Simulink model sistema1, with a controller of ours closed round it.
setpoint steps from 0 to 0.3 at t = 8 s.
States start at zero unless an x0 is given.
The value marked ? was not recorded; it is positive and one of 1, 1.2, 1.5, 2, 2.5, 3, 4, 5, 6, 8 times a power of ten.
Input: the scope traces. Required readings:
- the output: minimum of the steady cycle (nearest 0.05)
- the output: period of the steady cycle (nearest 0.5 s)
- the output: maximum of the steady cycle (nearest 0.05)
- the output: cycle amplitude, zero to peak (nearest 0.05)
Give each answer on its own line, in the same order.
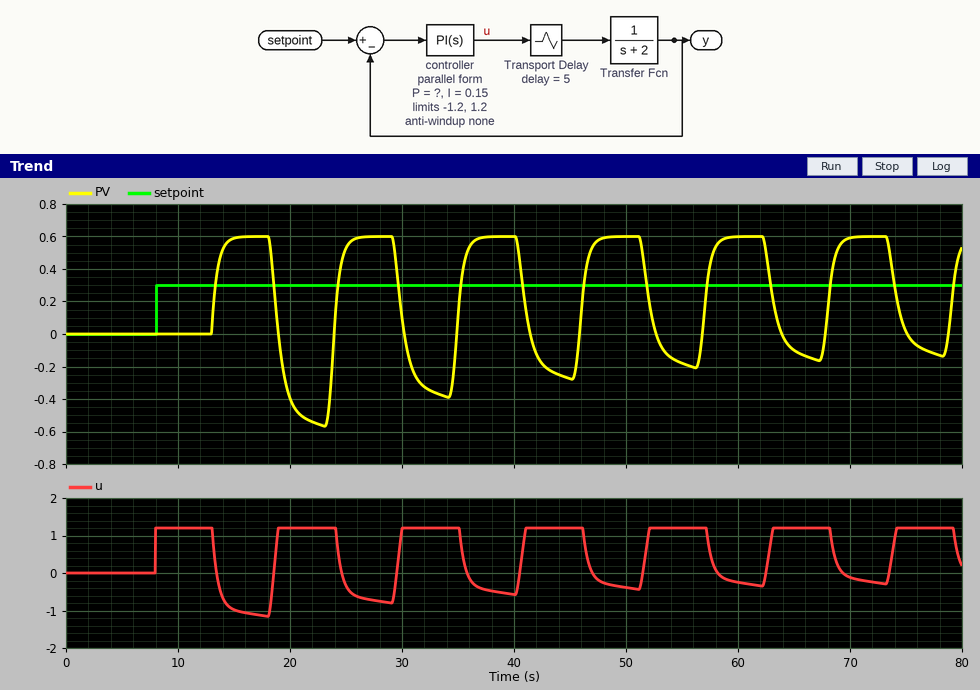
-0.40
11.0 s
0.60
0.50
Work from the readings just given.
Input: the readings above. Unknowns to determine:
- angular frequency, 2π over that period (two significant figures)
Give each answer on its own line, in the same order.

0.57 rad/s
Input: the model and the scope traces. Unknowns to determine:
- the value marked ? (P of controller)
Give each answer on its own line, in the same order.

4
